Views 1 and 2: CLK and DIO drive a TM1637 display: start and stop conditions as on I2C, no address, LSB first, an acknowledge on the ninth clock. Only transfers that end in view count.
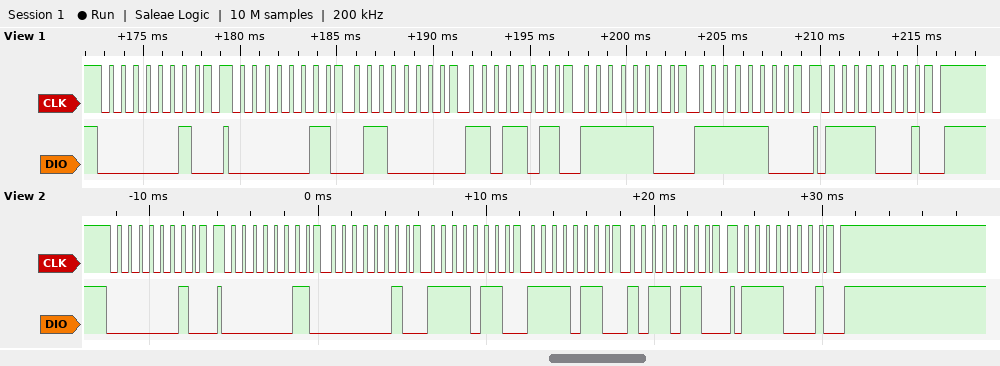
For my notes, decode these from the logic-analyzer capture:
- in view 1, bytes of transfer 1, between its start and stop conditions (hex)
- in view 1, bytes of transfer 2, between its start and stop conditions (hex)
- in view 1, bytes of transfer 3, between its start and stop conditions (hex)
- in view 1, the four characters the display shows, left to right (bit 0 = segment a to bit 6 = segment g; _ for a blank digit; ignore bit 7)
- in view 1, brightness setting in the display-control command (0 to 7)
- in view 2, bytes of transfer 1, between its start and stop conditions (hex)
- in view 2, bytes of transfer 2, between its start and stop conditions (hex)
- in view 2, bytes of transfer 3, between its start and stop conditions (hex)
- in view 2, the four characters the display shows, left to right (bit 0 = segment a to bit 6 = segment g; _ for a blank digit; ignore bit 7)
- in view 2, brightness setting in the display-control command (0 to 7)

40
C0 06 DB 3F 3F
8F
1200
7
40
C0 40 6F 6F 6D
8F
-995
7
